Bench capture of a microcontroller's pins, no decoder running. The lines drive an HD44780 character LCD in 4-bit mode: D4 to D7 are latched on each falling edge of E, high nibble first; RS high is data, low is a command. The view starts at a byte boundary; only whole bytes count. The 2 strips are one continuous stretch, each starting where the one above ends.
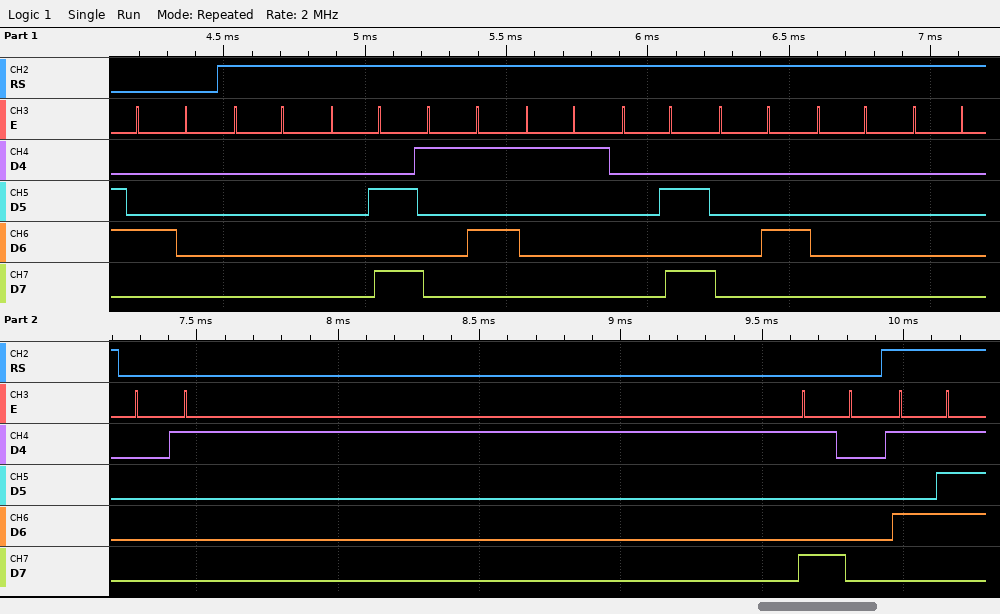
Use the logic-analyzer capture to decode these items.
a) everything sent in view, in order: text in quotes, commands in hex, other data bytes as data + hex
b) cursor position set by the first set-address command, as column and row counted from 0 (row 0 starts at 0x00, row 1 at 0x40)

0x40 data 00 0A 15 11 0A 04 00 00 0x01 0x90 "W"
column 16, row 0
